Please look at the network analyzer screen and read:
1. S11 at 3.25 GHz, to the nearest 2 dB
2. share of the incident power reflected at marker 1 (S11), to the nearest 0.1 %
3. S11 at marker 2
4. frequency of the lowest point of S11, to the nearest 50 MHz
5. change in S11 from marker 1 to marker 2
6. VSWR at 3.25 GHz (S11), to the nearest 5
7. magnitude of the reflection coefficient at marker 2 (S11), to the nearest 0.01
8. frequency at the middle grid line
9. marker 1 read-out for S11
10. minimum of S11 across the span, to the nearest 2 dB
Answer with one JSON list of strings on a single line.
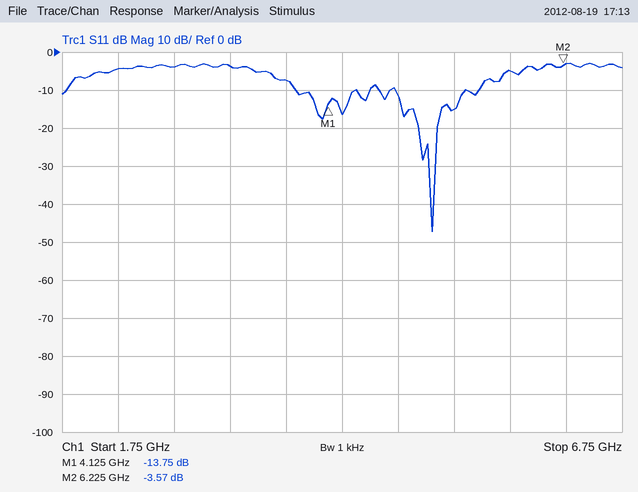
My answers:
["-4 dB", "4.2 %", "-3.57 dB", "5.05 GHz", "10.18 dB", "5", "0.66", "4.25 GHz", "-13.75 dB", "-48 dB"]
